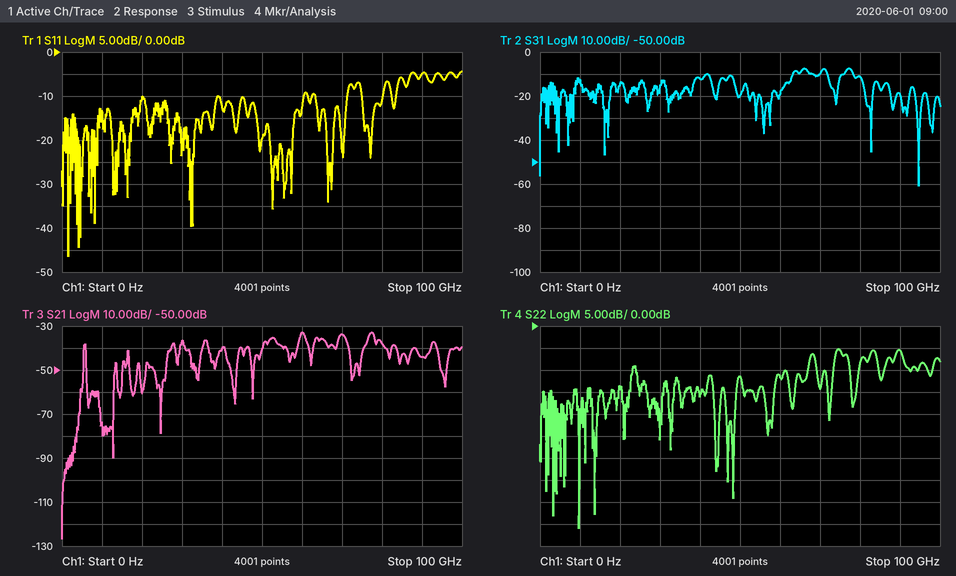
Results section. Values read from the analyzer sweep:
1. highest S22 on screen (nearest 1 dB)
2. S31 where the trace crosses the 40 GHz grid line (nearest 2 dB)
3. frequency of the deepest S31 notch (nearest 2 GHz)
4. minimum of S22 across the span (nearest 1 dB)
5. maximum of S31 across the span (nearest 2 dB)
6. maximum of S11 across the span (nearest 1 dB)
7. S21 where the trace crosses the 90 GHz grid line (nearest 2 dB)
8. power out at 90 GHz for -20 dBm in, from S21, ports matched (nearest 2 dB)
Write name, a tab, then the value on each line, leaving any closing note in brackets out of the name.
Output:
highest S22 on screen	-5 dB
S31 where the trace crosses the 40 GHz grid line	-12 dB
frequency of the deepest S31 notch	94 GHz
minimum of S22 across the span	-46 dB
maximum of S31 across the span	-8 dB
maximum of S11 across the span	-4 dB
S21 where the trace crosses the 90 GHz grid line	-44 dB
power out at 90 GHz for -20 dBm in, from S21, ports matched	-64 dBm
